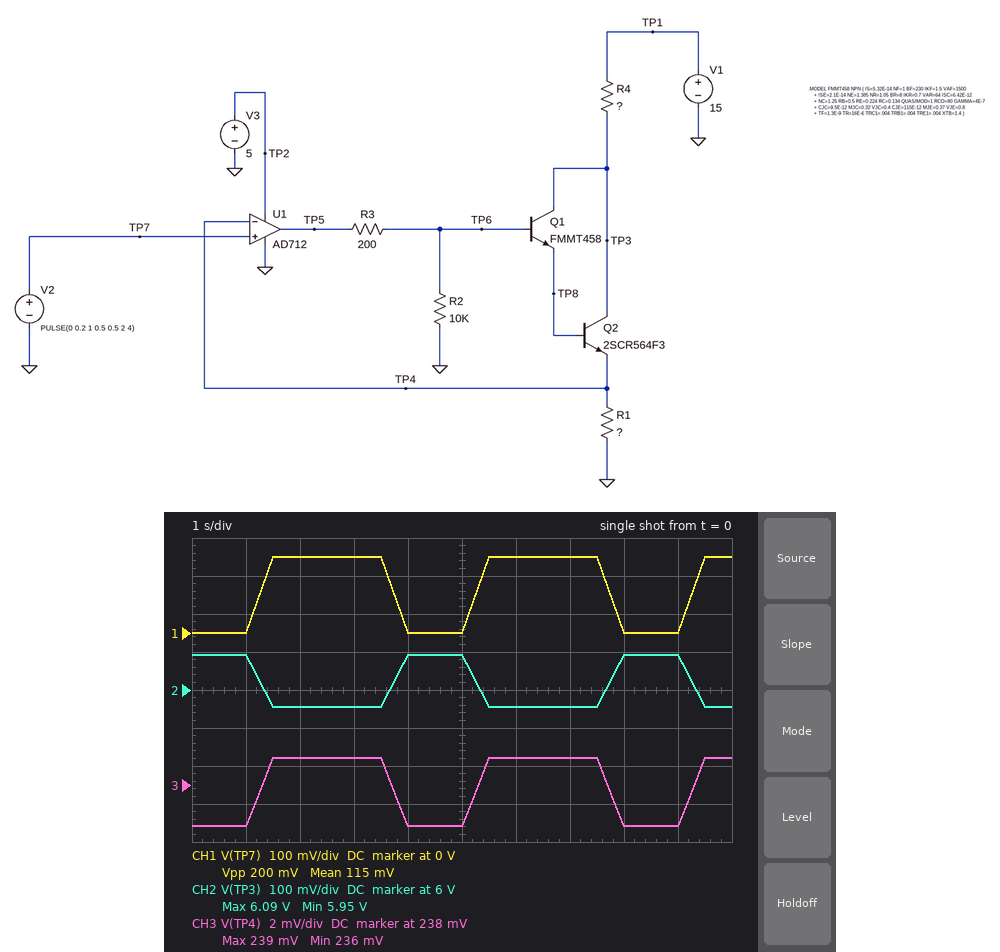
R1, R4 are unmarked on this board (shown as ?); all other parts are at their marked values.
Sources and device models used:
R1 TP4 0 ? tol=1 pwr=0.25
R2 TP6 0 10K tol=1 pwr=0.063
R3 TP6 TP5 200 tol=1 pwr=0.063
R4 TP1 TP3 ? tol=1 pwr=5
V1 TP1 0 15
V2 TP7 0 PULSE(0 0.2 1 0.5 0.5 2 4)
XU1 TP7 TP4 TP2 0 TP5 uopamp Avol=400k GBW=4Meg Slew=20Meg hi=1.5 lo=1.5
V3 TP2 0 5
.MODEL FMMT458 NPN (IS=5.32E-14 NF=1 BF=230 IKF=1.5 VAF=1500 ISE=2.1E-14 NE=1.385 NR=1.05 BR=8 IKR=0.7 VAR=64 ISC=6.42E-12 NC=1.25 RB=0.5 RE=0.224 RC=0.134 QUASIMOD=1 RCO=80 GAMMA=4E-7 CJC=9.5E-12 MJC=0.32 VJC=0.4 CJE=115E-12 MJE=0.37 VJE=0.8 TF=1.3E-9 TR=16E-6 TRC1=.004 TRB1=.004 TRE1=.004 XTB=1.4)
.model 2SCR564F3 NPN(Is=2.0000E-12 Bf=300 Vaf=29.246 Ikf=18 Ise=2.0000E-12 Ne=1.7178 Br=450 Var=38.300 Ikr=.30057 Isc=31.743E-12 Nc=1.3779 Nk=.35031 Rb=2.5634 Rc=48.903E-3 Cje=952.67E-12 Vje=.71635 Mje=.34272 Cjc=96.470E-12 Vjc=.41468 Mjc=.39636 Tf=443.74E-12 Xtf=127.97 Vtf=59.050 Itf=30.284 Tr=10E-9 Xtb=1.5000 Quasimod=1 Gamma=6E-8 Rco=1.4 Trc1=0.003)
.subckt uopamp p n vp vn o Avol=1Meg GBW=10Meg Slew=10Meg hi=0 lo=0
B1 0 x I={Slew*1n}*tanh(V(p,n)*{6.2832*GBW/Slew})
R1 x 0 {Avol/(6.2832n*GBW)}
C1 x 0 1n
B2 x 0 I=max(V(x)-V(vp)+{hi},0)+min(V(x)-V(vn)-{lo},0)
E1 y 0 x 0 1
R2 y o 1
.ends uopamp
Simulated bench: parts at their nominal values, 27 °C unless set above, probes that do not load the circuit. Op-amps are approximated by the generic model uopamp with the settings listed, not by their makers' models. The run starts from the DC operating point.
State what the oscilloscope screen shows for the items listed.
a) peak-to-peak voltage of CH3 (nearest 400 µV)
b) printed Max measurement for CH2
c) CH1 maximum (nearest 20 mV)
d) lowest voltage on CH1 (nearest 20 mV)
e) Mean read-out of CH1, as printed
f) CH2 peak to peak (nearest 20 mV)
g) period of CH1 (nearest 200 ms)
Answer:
3.6 mV
6.09 V
200 mV
0 V
115 mV
140 mV
4.0 s
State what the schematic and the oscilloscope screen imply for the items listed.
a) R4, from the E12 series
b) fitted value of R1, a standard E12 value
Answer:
68 Ω
1.8 Ω
